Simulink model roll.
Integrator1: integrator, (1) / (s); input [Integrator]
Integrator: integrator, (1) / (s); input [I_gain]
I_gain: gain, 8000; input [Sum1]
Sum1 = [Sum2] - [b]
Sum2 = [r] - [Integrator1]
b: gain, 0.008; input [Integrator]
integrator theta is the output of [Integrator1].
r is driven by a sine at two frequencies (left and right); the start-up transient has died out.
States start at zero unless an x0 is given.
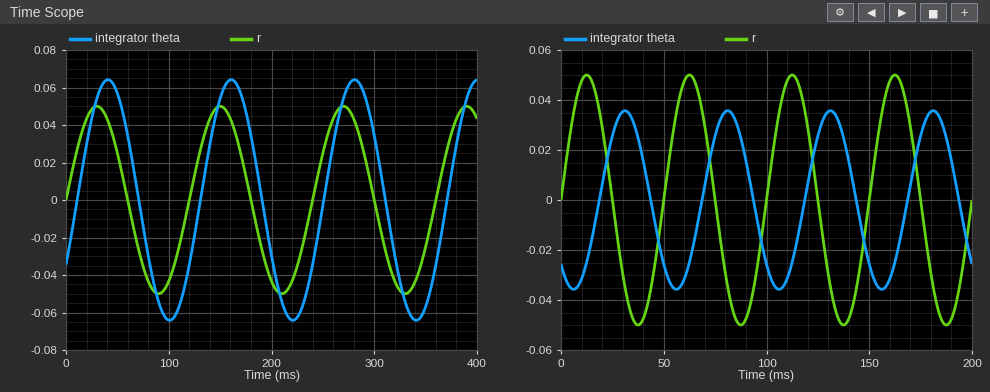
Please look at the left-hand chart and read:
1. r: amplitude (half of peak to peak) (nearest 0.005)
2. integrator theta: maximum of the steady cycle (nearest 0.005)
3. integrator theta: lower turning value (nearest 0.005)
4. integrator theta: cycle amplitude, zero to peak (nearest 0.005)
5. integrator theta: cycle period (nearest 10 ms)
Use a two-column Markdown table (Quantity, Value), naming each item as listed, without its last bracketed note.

| Quantity | Value |
|---|---|
| r: amplitude (half of peak to peak) | 0.050 |
| integrator theta: maximum of the steady cycle | 0.065 |
| integrator theta: lower turning value | -0.065 |
| integrator theta: cycle amplitude, zero to peak | 0.065 |
| integrator theta: cycle period | 120 ms |
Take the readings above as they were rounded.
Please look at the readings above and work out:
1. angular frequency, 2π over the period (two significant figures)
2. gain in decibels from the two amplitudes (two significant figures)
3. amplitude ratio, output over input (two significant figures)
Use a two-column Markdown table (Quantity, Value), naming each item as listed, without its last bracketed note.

| Quantity | Value |
|---|---|
| angular frequency, 2π over the period | 0.052 rad/ms |
| gain in decibels from the two amplitudes | 2.3 dB |
| amplitude ratio, output over input | 1.3 |
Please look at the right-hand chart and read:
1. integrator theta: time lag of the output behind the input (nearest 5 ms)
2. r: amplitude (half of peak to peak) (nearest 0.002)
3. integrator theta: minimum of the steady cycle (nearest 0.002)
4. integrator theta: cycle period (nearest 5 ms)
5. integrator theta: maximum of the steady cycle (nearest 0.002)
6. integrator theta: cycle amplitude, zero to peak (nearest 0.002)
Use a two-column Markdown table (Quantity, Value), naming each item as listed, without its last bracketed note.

| Quantity | Value |
|---|---|
| integrator theta: time lag of the output behind the input | 20 ms |
| r: amplitude (half of peak to peak) | 0.050 |
| integrator theta: minimum of the steady cycle | -0.036 |
| integrator theta: cycle period | 50 ms |
| integrator theta: maximum of the steady cycle | 0.036 |
| integrator theta: cycle amplitude, zero to peak | 0.036 |
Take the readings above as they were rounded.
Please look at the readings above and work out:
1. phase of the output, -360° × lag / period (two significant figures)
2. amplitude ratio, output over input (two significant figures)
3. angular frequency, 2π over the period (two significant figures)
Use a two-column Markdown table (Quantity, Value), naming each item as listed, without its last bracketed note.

| Quantity | Value |
|---|---|
| phase of the output, -360° × lag / period | -140° |
| amplitude ratio, output over input | 0.72 |
| angular frequency, 2π over the period | 0.13 rad/ms |
